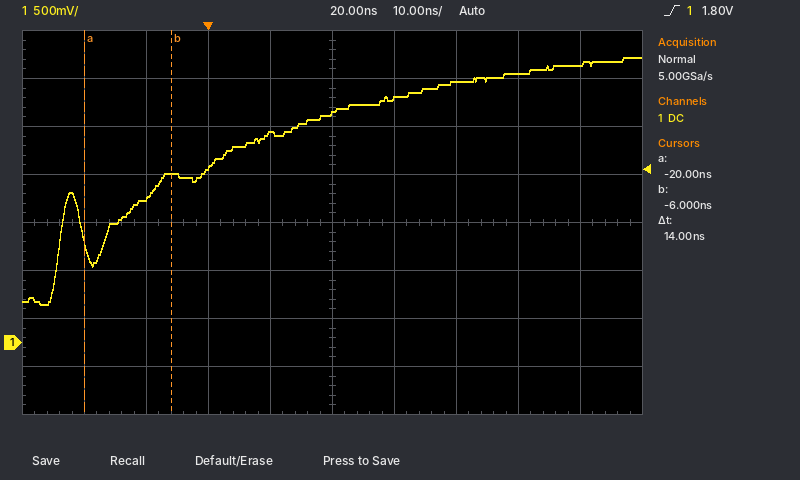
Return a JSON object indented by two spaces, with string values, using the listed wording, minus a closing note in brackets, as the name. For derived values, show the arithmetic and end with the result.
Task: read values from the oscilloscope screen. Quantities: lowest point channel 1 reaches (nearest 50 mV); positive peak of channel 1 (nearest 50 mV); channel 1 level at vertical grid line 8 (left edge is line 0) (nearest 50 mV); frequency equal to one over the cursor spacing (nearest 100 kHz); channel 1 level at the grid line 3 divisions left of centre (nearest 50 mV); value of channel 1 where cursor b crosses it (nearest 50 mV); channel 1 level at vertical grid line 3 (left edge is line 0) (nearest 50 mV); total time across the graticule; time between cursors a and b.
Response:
{
  "lowest point channel 1 reaches": "400 mV",
  "positive peak of channel 1": "2.95 V",
  "channel 1 level at vertical grid line 8 (left edge is line 0)": "2.80 V",
  "frequency equal to one over the cursor spacing": "1 / 14 ns ≈ 71.4 MHz",
  "channel 1 level at the grid line 3 divisions left of centre": "1.50 V",
  "value of channel 1 where cursor b crosses it": "1.75 V",
  "channel 1 level at vertical grid line 3 (left edge is line 0)": "1.80 V",
  "total time across the graticule": "100 ns",
  "time between cursors a and b": "14 ns"
}
